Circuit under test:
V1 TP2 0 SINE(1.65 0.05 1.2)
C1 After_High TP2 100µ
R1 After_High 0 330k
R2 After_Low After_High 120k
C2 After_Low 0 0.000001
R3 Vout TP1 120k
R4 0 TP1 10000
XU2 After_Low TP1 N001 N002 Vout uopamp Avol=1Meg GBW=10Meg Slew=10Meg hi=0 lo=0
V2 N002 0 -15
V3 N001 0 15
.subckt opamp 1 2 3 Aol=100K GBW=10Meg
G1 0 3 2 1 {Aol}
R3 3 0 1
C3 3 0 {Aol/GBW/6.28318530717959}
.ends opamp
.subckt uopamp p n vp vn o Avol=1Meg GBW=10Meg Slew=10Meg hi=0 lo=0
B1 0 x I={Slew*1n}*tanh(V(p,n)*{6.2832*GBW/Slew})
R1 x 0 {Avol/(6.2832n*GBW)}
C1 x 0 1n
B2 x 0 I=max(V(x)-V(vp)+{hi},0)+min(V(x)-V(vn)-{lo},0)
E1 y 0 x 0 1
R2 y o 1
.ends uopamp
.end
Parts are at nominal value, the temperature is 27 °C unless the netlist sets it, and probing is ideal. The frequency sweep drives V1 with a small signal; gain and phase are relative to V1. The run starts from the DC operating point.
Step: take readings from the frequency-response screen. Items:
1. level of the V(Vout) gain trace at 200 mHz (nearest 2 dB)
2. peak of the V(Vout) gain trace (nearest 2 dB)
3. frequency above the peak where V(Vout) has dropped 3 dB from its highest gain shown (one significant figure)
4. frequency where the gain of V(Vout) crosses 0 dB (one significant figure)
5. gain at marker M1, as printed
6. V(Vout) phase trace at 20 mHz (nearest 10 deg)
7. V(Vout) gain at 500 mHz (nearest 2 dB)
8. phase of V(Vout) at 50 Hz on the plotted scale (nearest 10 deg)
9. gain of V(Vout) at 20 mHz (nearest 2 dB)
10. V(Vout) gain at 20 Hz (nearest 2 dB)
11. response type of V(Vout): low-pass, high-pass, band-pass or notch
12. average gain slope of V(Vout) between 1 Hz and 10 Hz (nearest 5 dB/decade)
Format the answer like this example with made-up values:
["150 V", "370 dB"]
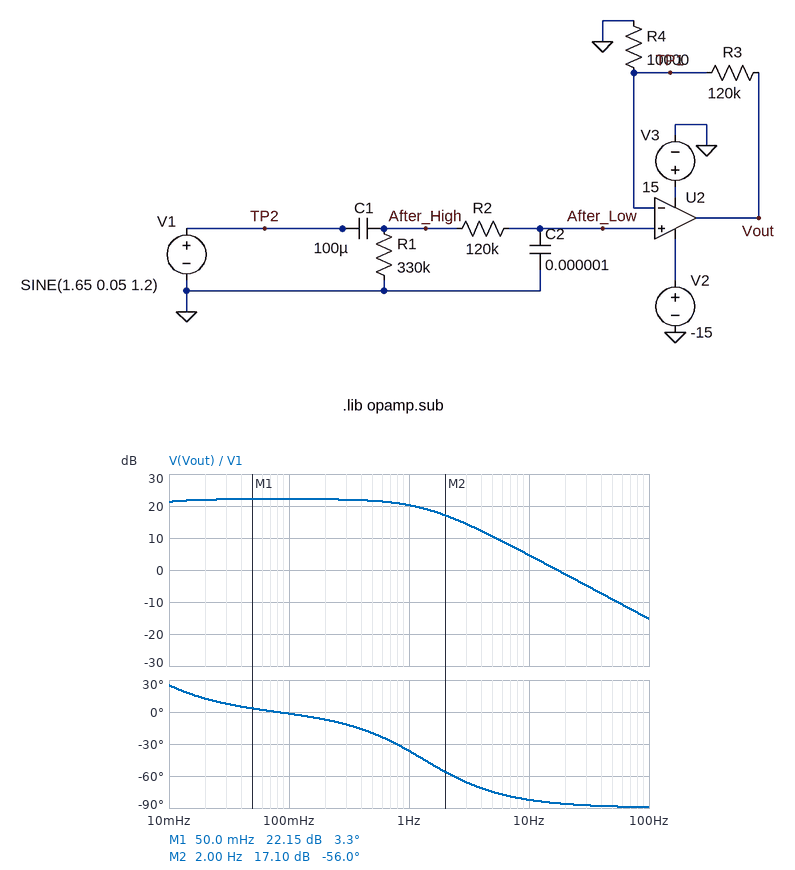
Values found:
["22 dB", "22 dB", "1 Hz", "20 Hz", "22.15 dB", "10 deg", "22 dB", "-90 deg", "22 dB", "-2 dB", "low-pass", "-15 dB/decade"]
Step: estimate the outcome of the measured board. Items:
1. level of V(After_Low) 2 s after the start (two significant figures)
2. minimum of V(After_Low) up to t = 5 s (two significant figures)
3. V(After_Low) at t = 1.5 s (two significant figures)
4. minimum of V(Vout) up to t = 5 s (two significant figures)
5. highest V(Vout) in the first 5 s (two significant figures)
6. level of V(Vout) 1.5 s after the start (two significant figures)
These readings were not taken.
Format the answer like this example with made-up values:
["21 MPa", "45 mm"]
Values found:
["36 mV", "-37 mV", "-34 mV", "-480 mV", "500 mV", "-440 mV"]
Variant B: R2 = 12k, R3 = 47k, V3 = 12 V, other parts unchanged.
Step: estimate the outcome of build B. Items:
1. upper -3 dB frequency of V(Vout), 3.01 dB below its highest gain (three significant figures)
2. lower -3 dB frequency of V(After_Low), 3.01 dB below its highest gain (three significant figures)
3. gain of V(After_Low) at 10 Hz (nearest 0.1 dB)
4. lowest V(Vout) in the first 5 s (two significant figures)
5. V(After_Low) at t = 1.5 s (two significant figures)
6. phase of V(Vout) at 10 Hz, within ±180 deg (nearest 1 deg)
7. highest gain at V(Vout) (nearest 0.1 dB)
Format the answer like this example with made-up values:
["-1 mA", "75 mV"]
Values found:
["13.4 Hz", "4.77 mHz", "-2.0 dB", "-280 mV", "-48 mV", "-37 deg", "15.0 dB"]
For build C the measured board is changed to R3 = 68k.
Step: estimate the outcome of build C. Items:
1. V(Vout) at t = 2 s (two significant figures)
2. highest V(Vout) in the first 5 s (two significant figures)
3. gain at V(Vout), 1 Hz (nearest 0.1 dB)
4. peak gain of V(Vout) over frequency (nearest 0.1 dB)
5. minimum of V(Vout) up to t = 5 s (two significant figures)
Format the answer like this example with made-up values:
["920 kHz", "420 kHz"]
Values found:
["280 mV", "300 mV", "15.8 dB", "17.7 dB", "-290 mV"]
